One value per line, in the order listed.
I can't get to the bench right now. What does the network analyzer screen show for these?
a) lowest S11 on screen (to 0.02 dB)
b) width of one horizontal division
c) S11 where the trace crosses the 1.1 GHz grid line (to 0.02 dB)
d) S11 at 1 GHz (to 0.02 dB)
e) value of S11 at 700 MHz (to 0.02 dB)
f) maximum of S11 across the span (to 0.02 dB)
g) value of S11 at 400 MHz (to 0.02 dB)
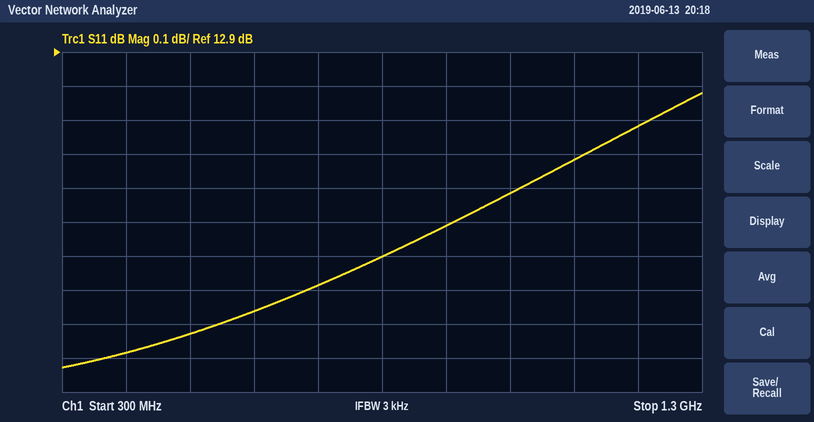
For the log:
11.98 dB
100 MHz
12.58 dB
12.48 dB
12.22 dB
12.78 dB
12.02 dB
